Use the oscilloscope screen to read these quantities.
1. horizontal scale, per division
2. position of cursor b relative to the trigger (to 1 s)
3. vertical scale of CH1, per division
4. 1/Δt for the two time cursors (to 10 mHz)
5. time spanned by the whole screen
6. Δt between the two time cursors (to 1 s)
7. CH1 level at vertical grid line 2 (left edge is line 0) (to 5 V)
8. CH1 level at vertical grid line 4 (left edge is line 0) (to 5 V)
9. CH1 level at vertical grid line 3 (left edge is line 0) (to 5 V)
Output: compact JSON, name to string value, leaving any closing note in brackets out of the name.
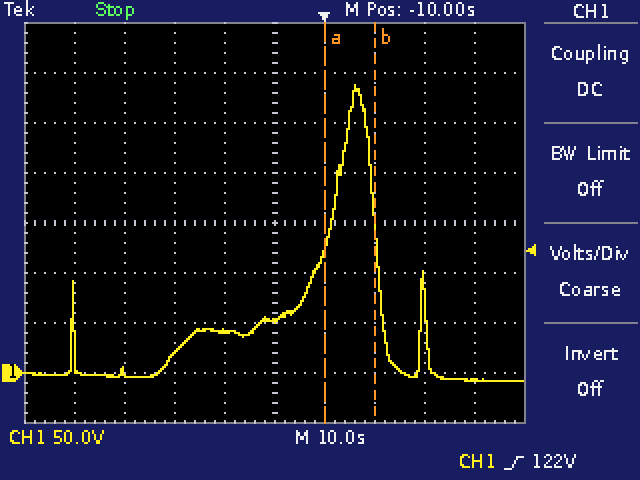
{"horizontal scale, per division": "10 s", "position of cursor b relative to the trigger": "+10 s", "vertical scale of CH1, per division": "50 V", "1/Δt for the two time cursors": "100 mHz", "time spanned by the whole screen": "100 s", "Δt between the two time cursors": "10 s", "CH1 level at vertical grid line 2 (left edge is line 0)": "0 V", "CH1 level at vertical grid line 4 (left edge is line 0)": "40 V", "CH1 level at vertical grid line 3 (left edge is line 0)": "20 V"}
